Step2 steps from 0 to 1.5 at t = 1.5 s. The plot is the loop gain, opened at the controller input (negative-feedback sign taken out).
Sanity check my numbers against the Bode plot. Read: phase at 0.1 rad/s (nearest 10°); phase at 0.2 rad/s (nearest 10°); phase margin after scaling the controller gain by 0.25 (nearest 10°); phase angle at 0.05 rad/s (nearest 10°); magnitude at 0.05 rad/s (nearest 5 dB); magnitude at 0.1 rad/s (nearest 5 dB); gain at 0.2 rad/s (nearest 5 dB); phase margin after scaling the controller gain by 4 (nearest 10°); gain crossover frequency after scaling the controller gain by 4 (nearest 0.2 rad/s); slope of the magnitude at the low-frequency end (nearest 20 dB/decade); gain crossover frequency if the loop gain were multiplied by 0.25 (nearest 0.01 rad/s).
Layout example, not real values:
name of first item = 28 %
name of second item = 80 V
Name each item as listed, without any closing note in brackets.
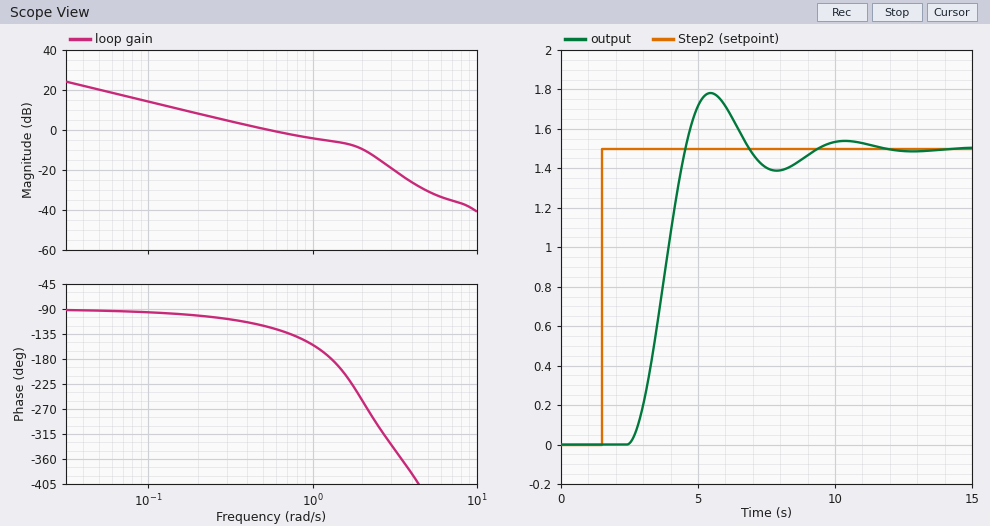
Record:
phase at 0.1 rad/s = -100°
phase at 0.2 rad/s = -100°
phase margin after scaling the controller gain by 0.25 = 80°
phase angle at 0.05 rad/s = -90°
magnitude at 0.05 rad/s = 20 dB
magnitude at 0.1 rad/s = 15 dB
gain at 0.2 rad/s = 10 dB
phase margin after scaling the controller gain by 4 = -100°
gain crossover frequency after scaling the controller gain by 4 = 2.2 rad/s
slope of the magnitude at the low-frequency end = -20 dB/decade
gain crossover frequency if the loop gain were multiplied by 0.25 = 0.13 rad/s
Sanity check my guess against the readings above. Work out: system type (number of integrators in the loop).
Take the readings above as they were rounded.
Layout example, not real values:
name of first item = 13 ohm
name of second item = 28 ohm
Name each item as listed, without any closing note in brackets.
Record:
system type = 1
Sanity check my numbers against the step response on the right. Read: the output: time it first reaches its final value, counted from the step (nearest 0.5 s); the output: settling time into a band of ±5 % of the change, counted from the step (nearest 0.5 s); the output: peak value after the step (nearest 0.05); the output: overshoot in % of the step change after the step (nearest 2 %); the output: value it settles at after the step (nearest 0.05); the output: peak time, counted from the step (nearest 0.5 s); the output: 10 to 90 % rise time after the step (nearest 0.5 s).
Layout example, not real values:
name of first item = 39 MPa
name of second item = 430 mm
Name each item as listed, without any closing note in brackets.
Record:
the output: time it first reaches its final value, counted from the step = 3.0 s
the output: settling time into a band of ±5 % of the change, counted from the step = 7.0 s
the output: peak value after the step = 1.80
the output: overshoot in % of the step change after the step = 18 %
the output: value it settles at after the step = 1.50
the output: peak time, counted from the step = 4.0 s
the output: 10 to 90 % rise time after the step = 1.5 s
